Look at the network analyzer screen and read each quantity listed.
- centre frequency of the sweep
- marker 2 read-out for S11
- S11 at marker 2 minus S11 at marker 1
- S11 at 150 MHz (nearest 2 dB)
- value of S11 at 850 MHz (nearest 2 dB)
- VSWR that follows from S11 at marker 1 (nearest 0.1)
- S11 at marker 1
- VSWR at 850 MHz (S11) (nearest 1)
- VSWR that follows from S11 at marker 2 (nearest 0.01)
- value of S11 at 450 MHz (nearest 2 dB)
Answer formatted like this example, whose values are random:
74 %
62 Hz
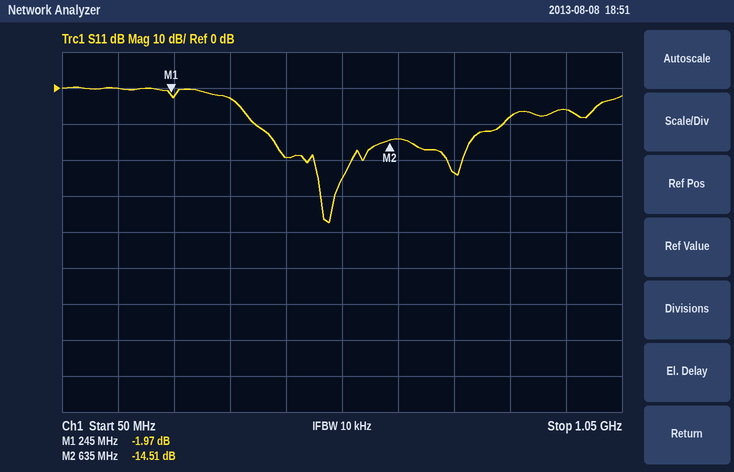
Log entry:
550 MHz
-14.51 dB
-12.54 dB
0 dB
-8 dB
8.9
-1.97 dB
2
1.46
-20 dB
